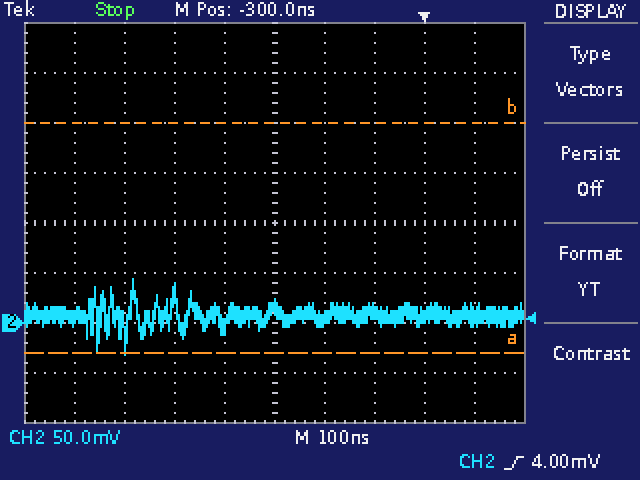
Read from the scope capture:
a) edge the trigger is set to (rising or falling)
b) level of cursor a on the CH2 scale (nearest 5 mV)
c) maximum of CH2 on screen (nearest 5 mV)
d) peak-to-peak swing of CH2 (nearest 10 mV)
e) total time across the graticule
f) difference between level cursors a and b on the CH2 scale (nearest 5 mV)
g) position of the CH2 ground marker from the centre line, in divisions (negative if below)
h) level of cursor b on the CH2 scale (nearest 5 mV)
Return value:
rising
-30 mV
45 mV
80 mV
1 µs
230 mV
-2.0 div
200 mV
